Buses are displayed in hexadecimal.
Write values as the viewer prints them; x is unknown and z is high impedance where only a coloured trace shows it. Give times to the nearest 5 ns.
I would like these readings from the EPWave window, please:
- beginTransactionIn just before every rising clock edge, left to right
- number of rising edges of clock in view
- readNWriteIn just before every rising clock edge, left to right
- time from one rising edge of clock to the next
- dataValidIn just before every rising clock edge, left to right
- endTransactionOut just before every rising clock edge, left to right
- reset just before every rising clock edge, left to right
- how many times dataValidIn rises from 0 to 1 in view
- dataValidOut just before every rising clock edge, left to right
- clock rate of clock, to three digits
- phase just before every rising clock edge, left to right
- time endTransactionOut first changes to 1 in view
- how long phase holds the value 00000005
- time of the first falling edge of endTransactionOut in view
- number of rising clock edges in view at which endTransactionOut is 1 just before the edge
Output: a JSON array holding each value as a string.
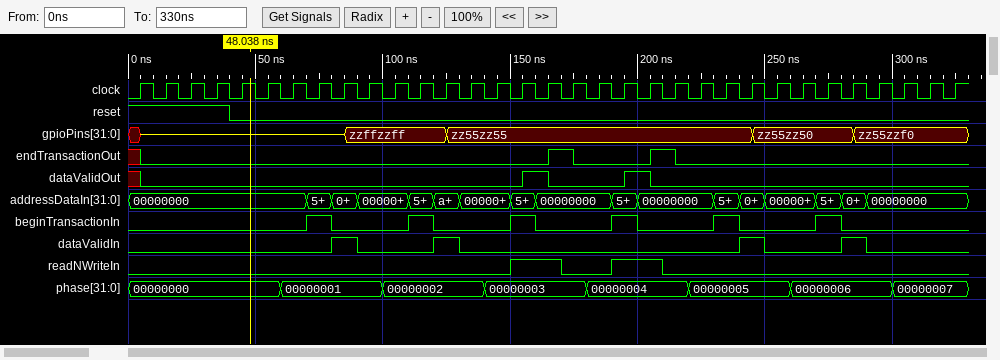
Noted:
["0 0 0 0 0 0 0 1 0 0 0 1 0 0 0 1 0 0 0 1 0 0 0 1 0 0 0 1 0 0 0 0 0", "33", "0 0 0 0 0 0 0 0 0 0 0 0 0 0 0 1 1 0 0 1 1 0 0 0 0 0 0 0 0 0 0 0 0", "10 ns", "0 0 0 0 0 0 0 0 1 0 0 0 1 0 0 0 0 0 0 0 0 0 0 0 1 0 0 0 1 0 0 0 0", "x 0 0 0 0 0 0 0 0 0 0 0 0 0 0 0 0 1 0 0 0 1 0 0 0 0 0 0 0 0 0 0 0", "1 1 1 1 0 0 0 0 0 0 0 0 0 0 0 0 0 0 0 0 0 0 0 0 0 0 0 0 0 0 0 0 0", "4", "x 0 0 0 0 0 0 0 0 0 0 0 0 0 0 0 1 0 0 0 1 0 0 0 0 0 0 0 0 0 0 0 0", "100 MHz", "00000000, 00000000, 00000000, 00000000, 00000000, 00000000, 00000001, 00000001, 00000001, 00000001, 00000002, 00000002, 00000002, 00000002, 00000003, 00000003, 00000003, 00000003, 00000004, 00000004, 00000004, 00000004, 00000005, 00000005, 00000005, 00000005, 00000006, 00000006, 00000006, 00000006, 00000007, 00000007, 00000007", "165 ns", "40 ns", "175 ns", "2"]
